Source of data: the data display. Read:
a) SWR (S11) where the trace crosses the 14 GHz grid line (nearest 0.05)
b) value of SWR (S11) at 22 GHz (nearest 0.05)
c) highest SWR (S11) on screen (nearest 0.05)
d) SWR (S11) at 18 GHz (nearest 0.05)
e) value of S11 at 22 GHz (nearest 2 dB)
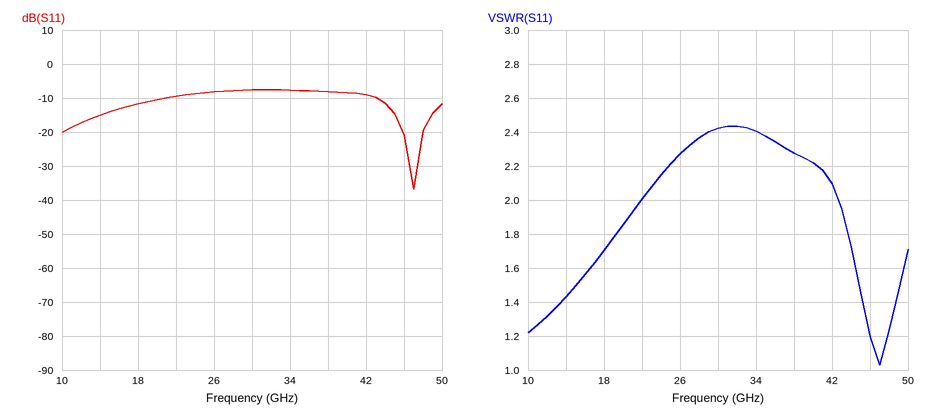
1.45
2.00
2.45
1.70
-10 dB
